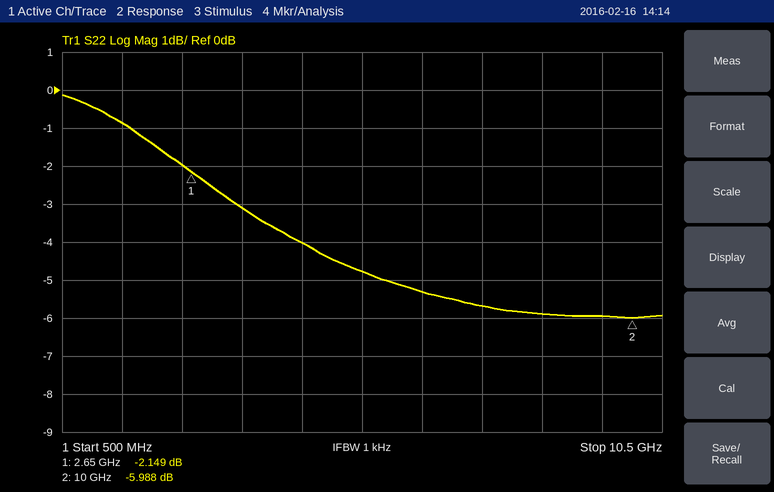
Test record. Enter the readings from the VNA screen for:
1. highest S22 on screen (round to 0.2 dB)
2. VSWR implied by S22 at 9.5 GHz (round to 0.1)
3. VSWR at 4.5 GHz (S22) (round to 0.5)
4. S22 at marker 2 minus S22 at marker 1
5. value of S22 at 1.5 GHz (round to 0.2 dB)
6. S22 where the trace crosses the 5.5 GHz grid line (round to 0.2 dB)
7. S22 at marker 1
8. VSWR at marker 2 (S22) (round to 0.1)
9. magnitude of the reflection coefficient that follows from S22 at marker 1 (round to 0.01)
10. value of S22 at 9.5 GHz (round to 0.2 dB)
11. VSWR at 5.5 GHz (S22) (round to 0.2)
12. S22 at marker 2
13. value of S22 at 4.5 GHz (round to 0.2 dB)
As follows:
-0.2 dB
3.0
4.5
-3.839 dB
-0.8 dB
-4.8 dB
-2.149 dB
3.0
0.78
-6.0 dB
3.8
-5.988 dB
-4.0 dB
